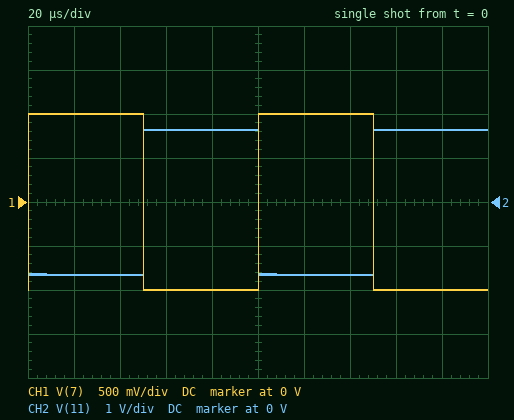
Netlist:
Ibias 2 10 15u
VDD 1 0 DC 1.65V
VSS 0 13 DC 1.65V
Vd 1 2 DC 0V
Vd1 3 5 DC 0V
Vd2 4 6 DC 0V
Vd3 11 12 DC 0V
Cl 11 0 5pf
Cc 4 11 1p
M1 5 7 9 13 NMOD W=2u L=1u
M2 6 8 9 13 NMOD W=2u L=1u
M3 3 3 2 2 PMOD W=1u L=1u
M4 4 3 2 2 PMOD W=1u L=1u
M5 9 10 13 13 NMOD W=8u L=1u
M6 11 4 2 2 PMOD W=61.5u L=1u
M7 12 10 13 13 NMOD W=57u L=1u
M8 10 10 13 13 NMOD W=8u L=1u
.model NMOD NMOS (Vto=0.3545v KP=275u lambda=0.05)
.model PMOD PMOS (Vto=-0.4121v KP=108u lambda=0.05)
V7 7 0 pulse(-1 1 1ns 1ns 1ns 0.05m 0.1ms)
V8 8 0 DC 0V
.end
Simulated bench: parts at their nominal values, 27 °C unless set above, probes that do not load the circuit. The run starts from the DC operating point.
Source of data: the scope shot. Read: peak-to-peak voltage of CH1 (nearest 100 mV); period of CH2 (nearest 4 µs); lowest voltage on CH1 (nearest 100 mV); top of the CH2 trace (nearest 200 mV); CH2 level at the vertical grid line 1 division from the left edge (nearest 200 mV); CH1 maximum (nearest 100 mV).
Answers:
2.0 V
100 µs
-1.0 V
1.6 V
-1.6 V
1.0 V
